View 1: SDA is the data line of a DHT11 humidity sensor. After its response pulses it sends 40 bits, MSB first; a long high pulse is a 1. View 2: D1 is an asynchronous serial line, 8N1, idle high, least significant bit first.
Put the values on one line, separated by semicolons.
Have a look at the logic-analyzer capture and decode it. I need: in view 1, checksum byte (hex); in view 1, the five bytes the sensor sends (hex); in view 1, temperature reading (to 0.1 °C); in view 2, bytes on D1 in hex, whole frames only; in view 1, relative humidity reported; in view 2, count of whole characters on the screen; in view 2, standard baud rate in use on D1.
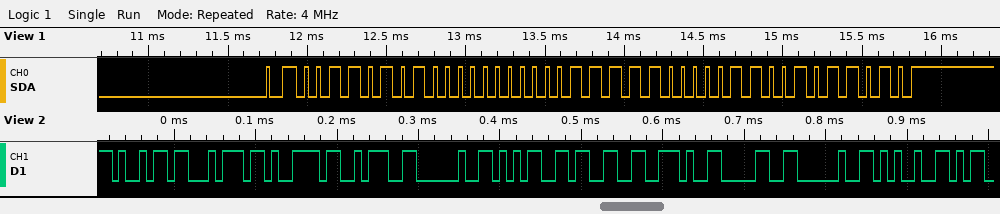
0x5A; 35 00 1F 06 5A; 31.6 °C; 69 74 79 3A 20 35 33 2E 30 20 25; 53 %; 11; 115200 baud
